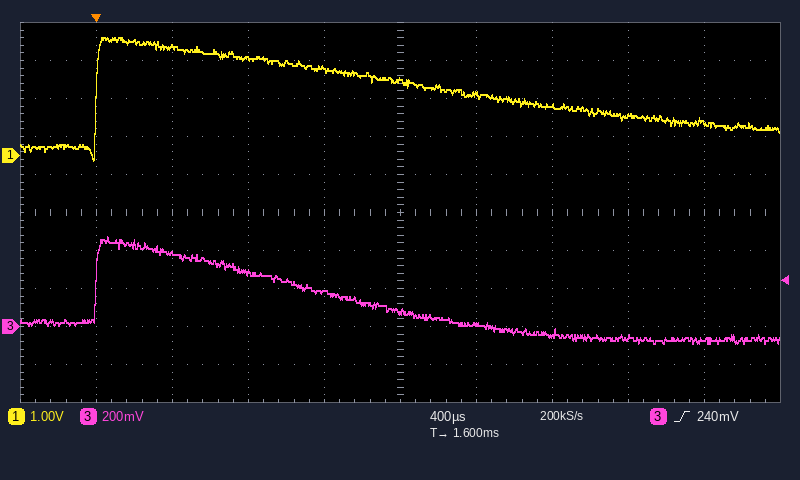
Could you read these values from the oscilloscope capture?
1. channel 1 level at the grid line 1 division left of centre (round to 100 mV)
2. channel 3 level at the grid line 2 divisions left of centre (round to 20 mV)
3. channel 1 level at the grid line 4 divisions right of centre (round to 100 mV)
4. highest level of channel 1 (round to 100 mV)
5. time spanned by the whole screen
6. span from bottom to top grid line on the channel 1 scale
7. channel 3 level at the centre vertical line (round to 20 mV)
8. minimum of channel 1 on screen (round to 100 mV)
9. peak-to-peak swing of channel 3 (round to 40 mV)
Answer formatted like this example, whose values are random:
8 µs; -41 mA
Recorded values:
2.3 V; 280 mV; 900 mV; 3.1 V; 4 ms; 10 V; 80 mV; -100 mV; 560 mV
